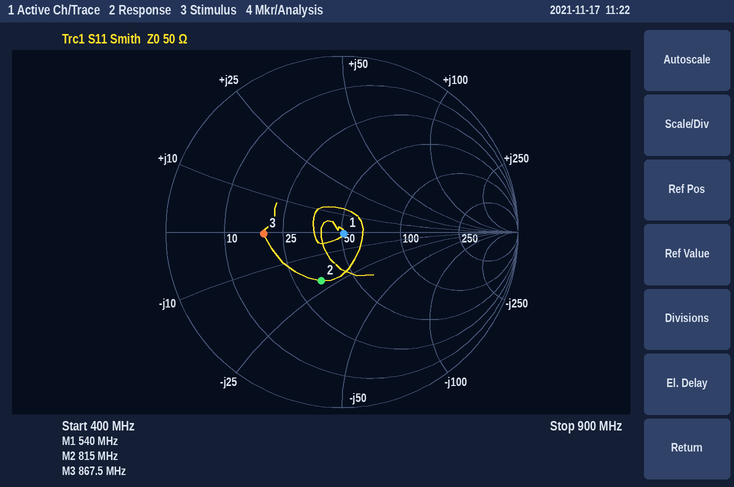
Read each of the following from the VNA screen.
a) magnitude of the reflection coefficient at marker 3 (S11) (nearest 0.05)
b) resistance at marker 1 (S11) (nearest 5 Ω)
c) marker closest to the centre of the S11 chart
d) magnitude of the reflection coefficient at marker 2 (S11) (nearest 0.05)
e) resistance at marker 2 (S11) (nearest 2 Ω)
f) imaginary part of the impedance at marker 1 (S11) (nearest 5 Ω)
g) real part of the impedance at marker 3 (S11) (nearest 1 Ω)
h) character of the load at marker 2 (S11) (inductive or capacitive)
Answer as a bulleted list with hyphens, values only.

- 0.45
- 50 Ω
- marker 1
- 0.30
- 34 Ω
- 0 Ω
- 19 Ω
- capacitive
